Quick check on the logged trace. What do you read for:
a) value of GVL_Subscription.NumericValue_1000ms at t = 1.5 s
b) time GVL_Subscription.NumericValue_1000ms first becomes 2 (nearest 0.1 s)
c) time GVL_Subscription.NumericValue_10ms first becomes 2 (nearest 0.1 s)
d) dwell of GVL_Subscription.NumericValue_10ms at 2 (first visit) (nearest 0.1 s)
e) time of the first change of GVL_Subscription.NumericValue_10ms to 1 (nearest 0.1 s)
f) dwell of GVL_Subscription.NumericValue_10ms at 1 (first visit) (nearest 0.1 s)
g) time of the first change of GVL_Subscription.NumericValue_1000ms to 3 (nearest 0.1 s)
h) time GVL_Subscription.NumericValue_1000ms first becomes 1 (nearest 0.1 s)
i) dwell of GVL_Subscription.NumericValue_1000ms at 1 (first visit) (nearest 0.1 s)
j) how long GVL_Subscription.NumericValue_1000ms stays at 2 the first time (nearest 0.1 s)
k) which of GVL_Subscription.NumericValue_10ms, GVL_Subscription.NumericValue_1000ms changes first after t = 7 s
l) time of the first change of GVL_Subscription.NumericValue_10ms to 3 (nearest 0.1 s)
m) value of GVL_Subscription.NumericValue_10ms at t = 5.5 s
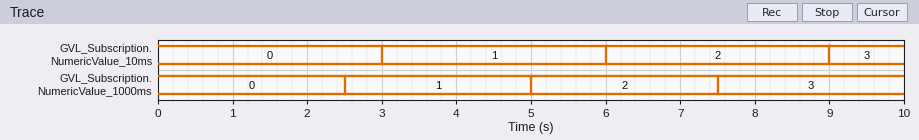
0
5.0 s
6.0 s
3.0 s
3.0 s
3.0 s
7.5 s
2.5 s
2.5 s
2.5 s
GVL_Subscription.NumericValue_1000ms
9.0 s
1
